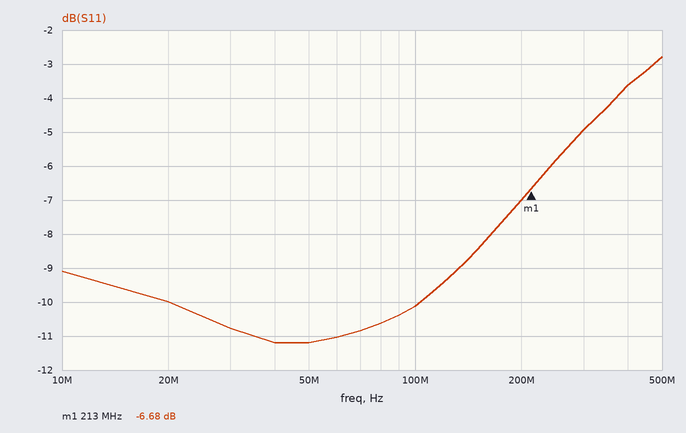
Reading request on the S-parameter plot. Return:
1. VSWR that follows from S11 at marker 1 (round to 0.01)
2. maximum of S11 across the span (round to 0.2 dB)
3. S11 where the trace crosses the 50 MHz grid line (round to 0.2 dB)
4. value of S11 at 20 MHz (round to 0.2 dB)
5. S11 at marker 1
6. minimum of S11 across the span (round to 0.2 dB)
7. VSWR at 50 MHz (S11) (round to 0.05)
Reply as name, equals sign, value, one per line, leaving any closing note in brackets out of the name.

VSWR that follows from S11 at marker 1 = 2.73
maximum of S11 across the span = -2.8 dB
S11 where the trace crosses the 50 MHz grid line = -11.2 dB
value of S11 at 20 MHz = -10.0 dB
S11 at marker 1 = -6.68 dB
minimum of S11 across the span = -11.2 dB
VSWR at 50 MHz (S11) = 1.75
